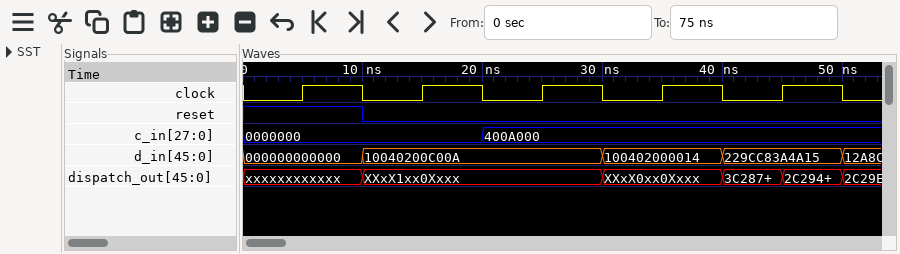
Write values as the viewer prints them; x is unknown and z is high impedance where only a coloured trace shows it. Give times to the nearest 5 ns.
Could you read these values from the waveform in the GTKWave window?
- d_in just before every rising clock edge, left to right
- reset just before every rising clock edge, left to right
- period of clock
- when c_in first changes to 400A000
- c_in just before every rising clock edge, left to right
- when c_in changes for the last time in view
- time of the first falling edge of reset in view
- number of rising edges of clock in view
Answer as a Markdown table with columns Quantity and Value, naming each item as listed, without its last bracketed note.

| Quantity | Value |
|---|---|
| d_in just before every rising clock edge, left to right | 000000000000, 10040200C00A, 10040200C00A, 100402000014, 229CC83A4A15 |
| reset just before every rising clock edge, left to right | 1 0 0 0 0 |
| period of clock | 10 ns |
| when c_in first changes to 400A000 | 20 ns |
| c_in just before every rising clock edge, left to right | 0000000, 0000000, 400A000, 400A000, 400A000 |
| when c_in changes for the last time in view | 20 ns |
| time of the first falling edge of reset in view | 10 ns |
| number of rising edges of clock in view | 5 |
